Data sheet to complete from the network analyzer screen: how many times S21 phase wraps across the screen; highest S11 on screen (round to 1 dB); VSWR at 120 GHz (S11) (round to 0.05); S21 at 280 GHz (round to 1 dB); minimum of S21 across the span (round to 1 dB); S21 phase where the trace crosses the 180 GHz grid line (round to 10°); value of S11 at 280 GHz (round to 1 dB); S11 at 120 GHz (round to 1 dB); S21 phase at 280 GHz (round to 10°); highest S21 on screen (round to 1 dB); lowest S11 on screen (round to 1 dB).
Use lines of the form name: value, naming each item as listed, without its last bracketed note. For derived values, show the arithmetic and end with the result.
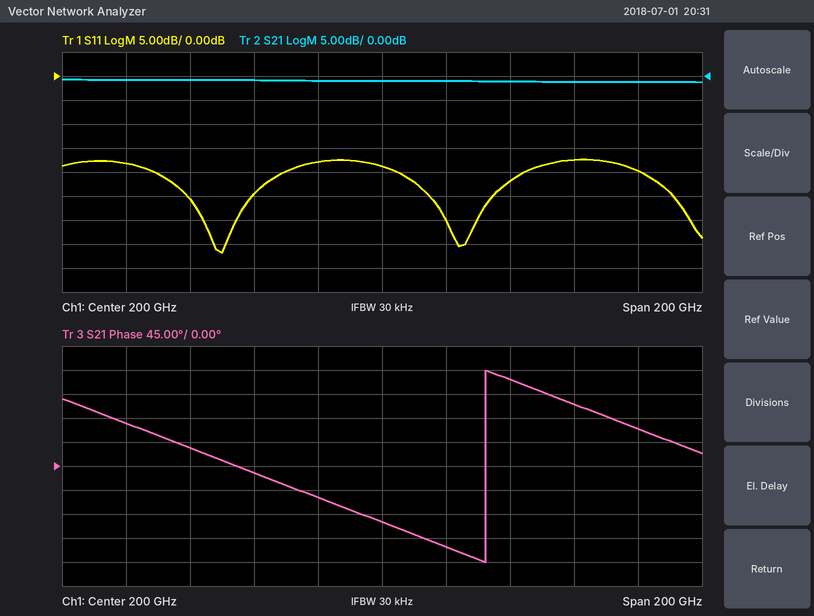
how many times S21 phase wraps across the screen: 1
highest S11 on screen: -17 dB
VSWR at 120 GHz (S11): |Γ| = 10^(-18/20) = 0.1259; VSWR = (1 + 0.1259)/(1 − 0.1259) ≈ 1.29, so 1.30 to the nearest 0.05
S21 at 280 GHz: -1 dB
minimum of S21 across the span: -1 dB
S21 phase where the trace crosses the 180 GHz grid line: -60°
value of S11 at 280 GHz: -20 dB
S11 at 120 GHz: -18 dB
S21 phase at 280 GHz: 70°
highest S21 on screen: -1 dB
lowest S11 on screen: -37 dB
